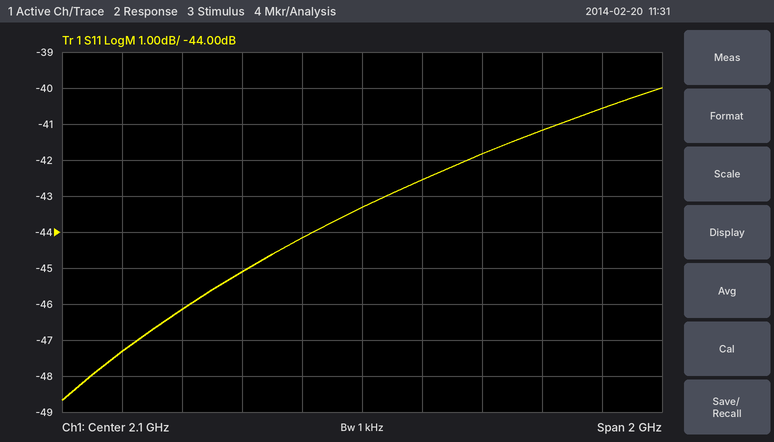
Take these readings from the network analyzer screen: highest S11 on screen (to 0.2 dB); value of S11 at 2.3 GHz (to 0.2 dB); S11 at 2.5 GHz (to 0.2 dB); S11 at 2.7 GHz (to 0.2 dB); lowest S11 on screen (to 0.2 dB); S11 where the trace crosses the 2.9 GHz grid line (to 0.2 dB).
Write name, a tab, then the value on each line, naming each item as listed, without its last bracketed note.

highest S11 on screen	-40.0 dB
value of S11 at 2.3 GHz	-42.6 dB
S11 at 2.5 GHz	-41.8 dB
S11 at 2.7 GHz	-41.2 dB
lowest S11 on screen	-48.6 dB
S11 where the trace crosses the 2.9 GHz grid line	-40.6 dB
